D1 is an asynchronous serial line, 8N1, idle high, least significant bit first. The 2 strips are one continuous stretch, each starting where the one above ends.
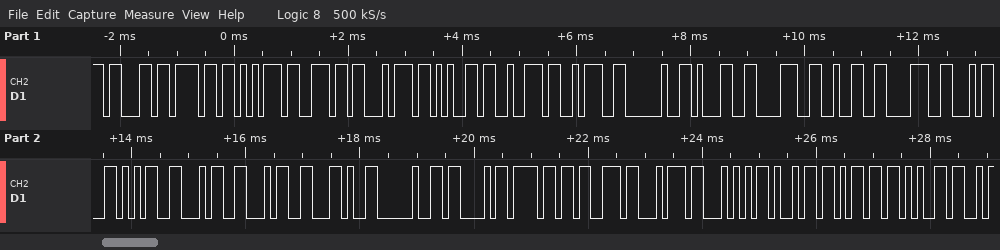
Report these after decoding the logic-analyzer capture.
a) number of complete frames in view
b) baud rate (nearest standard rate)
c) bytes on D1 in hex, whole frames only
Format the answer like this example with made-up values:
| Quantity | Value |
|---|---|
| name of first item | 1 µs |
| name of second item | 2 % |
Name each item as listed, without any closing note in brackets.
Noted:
| Quantity | Value |
|---|---|
| number of complete frames in view | 27 |
| baud rate | 9600 baud |
| bytes on D1 in hex, whole frames only | 63 6F 75 6E 74 65 72 3A 20 31 38 32 38 34 35 34 34 2C 20 43 6F 73 74 54 69 6D 65 |
